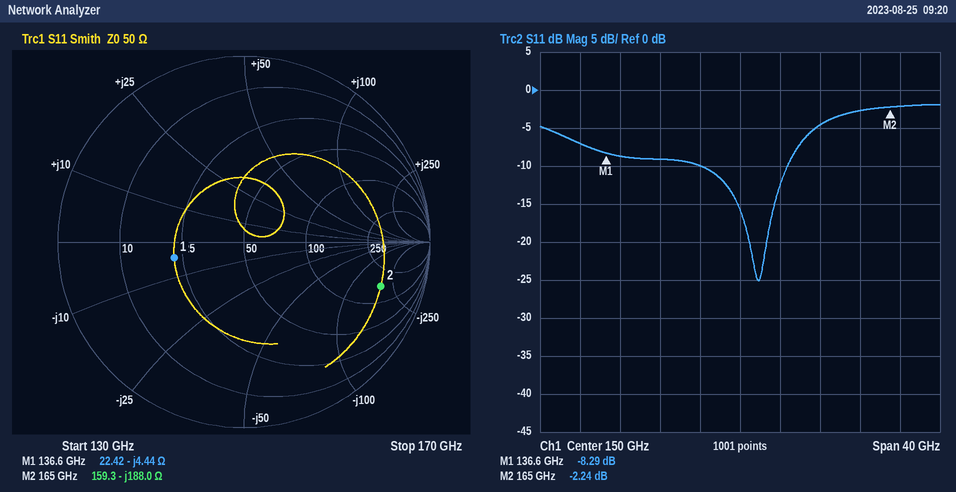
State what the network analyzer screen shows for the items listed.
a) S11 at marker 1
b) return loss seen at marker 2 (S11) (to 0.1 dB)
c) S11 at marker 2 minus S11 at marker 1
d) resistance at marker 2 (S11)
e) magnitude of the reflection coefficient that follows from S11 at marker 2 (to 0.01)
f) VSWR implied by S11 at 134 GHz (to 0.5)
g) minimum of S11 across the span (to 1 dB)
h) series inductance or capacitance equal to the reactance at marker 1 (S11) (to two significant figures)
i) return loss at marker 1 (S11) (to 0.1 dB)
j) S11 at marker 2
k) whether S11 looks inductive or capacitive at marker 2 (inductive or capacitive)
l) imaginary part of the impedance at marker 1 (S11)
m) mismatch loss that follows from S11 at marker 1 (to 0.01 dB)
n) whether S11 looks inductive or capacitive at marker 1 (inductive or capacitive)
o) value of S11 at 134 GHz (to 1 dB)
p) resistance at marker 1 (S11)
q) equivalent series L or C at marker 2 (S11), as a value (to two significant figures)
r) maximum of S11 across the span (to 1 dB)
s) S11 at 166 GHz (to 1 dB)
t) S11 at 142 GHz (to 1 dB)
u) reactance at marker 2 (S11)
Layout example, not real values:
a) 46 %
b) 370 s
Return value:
a) -8.29 dB
b) 2.2 dB
c) 6.05 dB
d) 159.3 Ω
e) 0.77
f) 2.5
g) -25 dB
h) 260 fF
i) 8.3 dB
j) -2.24 dB
k) capacitive
l) -4.44 Ω
m) 0.70 dB
n) capacitive
o) -7 dB
p) 22.42 Ω
q) 5.1 fF
r) -2 dB
s) -2 dB
t) -9 dB
u) -188.0 Ω
